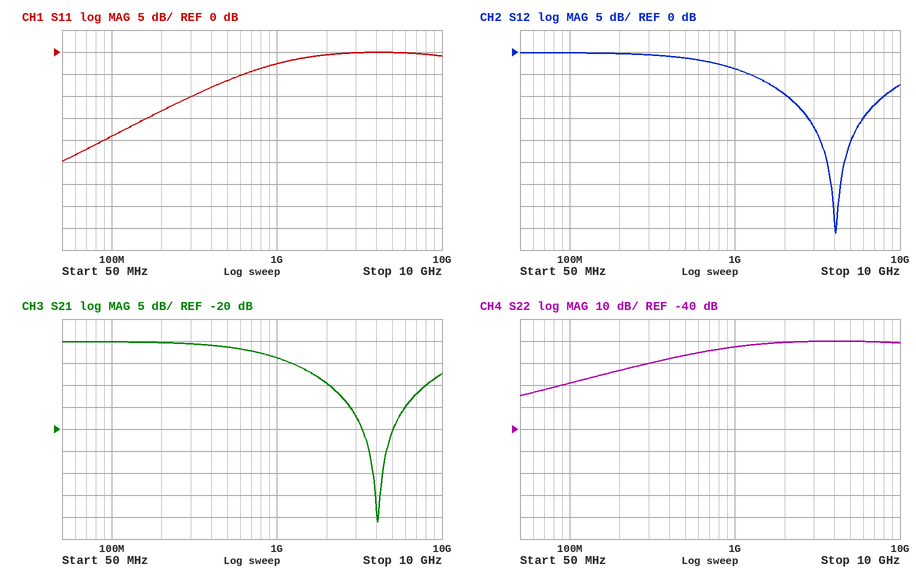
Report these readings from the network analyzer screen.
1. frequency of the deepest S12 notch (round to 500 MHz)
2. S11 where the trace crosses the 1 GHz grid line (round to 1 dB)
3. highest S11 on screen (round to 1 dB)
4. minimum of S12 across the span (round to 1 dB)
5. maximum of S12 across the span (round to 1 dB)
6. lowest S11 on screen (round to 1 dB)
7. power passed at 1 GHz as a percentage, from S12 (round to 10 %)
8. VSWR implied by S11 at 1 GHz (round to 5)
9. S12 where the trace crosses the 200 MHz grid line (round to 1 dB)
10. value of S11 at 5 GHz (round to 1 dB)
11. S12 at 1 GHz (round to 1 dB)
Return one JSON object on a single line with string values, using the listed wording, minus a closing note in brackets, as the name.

{"frequency of the deepest S12 notch": "4.0 GHz", "S11 where the trace crosses the 1 GHz grid line": "-3 dB", "highest S11 on screen": "0 dB", "minimum of S12 across the span": "-41 dB", "maximum of S12 across the span": "0 dB", "lowest S11 on screen": "-25 dB", "power passed at 1 GHz as a percentage, from S12": "40 %", "VSWR implied by S11 at 1 GHz": "5", "S12 where the trace crosses the 200 MHz grid line": "0 dB", "value of S11 at 5 GHz": "0 dB", "S12 at 1 GHz": "-4 dB"}
